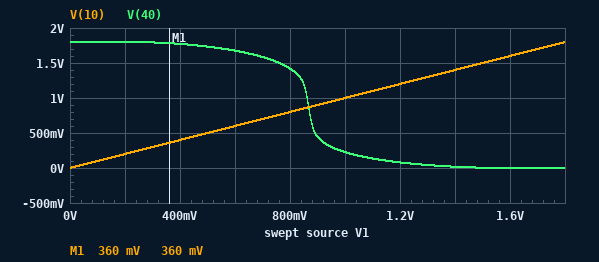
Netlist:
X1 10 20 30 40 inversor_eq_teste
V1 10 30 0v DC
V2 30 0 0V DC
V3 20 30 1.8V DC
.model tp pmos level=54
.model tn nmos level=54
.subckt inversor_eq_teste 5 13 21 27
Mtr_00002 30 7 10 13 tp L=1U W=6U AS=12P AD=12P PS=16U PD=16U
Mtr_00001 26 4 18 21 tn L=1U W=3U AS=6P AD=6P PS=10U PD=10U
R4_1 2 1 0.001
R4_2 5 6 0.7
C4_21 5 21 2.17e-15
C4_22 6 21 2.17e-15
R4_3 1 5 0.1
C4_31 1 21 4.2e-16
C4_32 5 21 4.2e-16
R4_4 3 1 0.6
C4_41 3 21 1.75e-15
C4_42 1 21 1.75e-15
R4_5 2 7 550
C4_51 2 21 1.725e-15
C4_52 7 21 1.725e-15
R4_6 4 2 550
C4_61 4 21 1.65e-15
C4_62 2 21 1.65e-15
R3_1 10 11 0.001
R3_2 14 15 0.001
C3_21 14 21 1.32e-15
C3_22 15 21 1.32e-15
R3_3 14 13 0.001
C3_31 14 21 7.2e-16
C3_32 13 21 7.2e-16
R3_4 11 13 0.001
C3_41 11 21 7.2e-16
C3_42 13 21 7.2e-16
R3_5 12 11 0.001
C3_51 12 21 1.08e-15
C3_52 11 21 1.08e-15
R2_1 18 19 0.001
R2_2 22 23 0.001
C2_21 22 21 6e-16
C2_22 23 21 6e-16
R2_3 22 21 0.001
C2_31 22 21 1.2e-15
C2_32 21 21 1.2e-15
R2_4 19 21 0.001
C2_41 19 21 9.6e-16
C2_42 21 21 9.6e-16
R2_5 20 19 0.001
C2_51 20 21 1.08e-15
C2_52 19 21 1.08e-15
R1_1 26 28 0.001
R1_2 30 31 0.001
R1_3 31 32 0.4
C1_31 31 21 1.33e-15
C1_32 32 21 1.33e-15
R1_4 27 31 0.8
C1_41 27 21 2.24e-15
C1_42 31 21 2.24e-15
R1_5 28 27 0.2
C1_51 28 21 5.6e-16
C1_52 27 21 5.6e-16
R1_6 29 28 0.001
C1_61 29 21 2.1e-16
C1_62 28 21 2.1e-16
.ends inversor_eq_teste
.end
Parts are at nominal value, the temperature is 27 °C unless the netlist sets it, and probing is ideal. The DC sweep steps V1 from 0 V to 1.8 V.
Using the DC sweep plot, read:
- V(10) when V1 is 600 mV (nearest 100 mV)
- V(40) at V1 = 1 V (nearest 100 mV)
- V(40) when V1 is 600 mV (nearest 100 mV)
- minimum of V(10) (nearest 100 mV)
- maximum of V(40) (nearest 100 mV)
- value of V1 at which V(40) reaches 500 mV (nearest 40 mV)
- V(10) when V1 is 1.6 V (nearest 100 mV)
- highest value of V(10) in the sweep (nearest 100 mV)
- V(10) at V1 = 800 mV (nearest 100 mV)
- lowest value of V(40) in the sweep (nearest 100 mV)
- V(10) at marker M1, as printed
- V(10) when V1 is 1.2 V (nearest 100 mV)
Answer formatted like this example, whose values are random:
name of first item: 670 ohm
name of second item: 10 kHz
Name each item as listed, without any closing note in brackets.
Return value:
V(10) when V1 is 600 mV: 600 mV
V(40) at V1 = 1 V: 200 mV
V(40) when V1 is 600 mV: 1.7 V
minimum of V(10): 0 V
maximum of V(40): 1.8 V
value of V1 at which V(40) reaches 500 mV: 880 mV
V(10) when V1 is 1.6 V: 1.6 V
highest value of V(10) in the sweep: 1.8 V
V(10) at V1 = 800 mV: 800 mV
lowest value of V(40) in the sweep: 0 V
V(10) at marker M1, as printed: 360 mV
V(10) when V1 is 1.2 V: 1.2 V
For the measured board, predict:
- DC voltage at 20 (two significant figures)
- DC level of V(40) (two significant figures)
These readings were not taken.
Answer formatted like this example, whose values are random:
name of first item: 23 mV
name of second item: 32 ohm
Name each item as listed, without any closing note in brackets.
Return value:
DC voltage at 20: 1.8 V
DC level of V(40): 1.8 V
